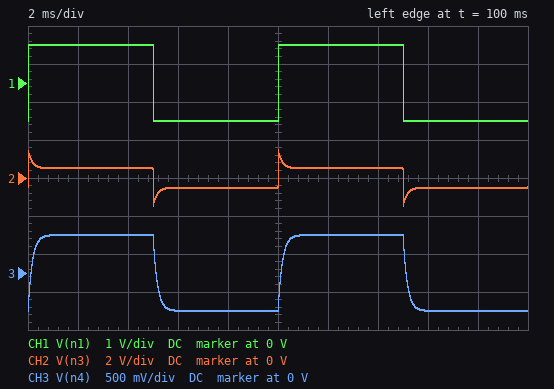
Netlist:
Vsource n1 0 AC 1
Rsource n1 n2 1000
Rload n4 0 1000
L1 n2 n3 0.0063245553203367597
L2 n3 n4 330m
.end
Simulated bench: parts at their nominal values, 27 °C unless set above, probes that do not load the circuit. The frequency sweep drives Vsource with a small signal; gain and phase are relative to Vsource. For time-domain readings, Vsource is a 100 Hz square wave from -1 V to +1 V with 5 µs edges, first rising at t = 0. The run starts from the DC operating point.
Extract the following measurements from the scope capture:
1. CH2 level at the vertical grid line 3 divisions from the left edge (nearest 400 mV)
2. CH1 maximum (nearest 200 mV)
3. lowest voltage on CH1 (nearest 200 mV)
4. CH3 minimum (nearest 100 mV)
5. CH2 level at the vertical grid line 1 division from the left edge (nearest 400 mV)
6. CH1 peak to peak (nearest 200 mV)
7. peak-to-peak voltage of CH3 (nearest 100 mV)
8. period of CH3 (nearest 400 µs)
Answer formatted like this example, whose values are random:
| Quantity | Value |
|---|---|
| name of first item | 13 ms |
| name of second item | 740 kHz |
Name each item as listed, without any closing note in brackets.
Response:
| Quantity | Value |
|---|---|
| CH2 level at the vertical grid line 3 divisions from the left edge | -400 mV |
| CH1 maximum | 1.0 V |
| lowest voltage on CH1 | -1.0 V |
| CH3 minimum | -500 mV |
| CH2 level at the vertical grid line 1 division from the left edge | 400 mV |
| CH1 peak to peak | 2.0 V |
| peak-to-peak voltage of CH3 | 1.0 V |
| period of CH3 | 10.0 ms |
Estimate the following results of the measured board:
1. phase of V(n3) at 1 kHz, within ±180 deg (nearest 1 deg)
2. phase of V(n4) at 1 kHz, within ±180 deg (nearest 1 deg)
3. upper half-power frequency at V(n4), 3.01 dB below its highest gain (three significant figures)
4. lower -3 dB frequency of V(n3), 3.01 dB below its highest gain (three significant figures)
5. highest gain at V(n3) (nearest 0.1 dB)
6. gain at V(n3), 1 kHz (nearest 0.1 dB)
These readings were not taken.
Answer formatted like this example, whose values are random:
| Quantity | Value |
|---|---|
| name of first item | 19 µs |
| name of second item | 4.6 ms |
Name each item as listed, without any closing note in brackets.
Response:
| Quantity | Value |
|---|---|
| phase of V(n3) at 1 kHz, within ±180 deg | 18 deg |
| phase of V(n4) at 1 kHz, within ±180 deg | -47 deg |
| upper half-power frequency at V(n4), 3.01 dB below its highest gain | 946 Hz |
| lower -3 dB frequency of V(n3), 3.01 dB below its highest gain | 656 Hz |
| highest gain at V(n3) | -0.2 dB |
| gain at V(n3), 1 kHz | -2.0 dB |
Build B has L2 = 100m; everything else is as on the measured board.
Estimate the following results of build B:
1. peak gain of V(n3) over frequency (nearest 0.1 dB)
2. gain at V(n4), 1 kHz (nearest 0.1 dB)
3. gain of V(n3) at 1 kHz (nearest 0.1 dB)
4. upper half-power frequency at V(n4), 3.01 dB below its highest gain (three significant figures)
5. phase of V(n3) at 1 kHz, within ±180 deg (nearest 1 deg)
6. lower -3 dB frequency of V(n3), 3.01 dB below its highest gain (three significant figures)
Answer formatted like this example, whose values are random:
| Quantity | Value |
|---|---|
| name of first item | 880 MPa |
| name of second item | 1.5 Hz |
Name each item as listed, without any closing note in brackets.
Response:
| Quantity | Value |
|---|---|
| peak gain of V(n3) over frequency | -0.5 dB |
| gain at V(n4), 1 kHz | -6.5 dB |
| gain of V(n3) at 1 kHz | -5.0 dB |
| upper half-power frequency at V(n4), 3.01 dB below its highest gain | 2.99 kHz |
| phase of V(n3) at 1 kHz, within ±180 deg | 14 deg |
| lower -3 dB frequency of V(n3), 3.01 dB below its highest gain | 1.97 kHz |
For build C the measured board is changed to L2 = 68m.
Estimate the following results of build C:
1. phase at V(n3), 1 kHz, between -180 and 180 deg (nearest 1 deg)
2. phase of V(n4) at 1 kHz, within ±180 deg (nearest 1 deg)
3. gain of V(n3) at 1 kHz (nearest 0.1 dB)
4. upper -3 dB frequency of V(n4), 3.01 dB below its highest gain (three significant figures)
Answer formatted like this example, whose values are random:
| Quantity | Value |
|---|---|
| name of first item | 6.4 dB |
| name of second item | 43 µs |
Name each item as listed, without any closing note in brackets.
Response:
| Quantity | Value |
|---|---|
| phase at V(n3), 1 kHz, between -180 and 180 deg | 10 deg |
| phase of V(n4) at 1 kHz, within ±180 deg | -13 deg |
| gain of V(n3) at 1 kHz | -5.5 dB |
| upper -3 dB frequency of V(n4), 3.01 dB below its highest gain | 4.28 kHz |
